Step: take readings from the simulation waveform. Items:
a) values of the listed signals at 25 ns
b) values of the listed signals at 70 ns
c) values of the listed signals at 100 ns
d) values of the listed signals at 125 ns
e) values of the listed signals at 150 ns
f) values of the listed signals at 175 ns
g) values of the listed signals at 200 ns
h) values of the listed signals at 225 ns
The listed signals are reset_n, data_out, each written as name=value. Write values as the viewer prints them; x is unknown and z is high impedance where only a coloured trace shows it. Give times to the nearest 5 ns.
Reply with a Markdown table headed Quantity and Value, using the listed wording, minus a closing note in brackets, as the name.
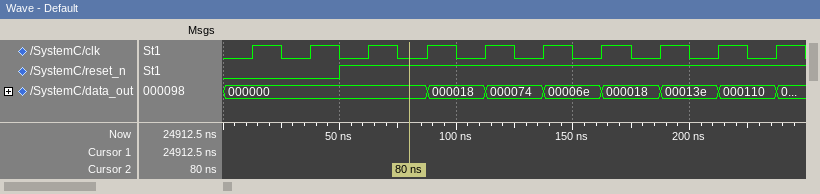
| Quantity | Value |
|---|---|
| values of the listed signals at 25 ns | reset_n=0, data_out=000000 |
| values of the listed signals at 70 ns | reset_n=1, data_out=000000 |
| values of the listed signals at 100 ns | reset_n=1, data_out=000018 |
| values of the listed signals at 125 ns | reset_n=1, data_out=000074 |
| values of the listed signals at 150 ns | reset_n=1, data_out=00006e |
| values of the listed signals at 175 ns | reset_n=1, data_out=000018 |
| values of the listed signals at 200 ns | reset_n=1, data_out=00013e |
| values of the listed signals at 225 ns | reset_n=1, data_out=000110 |
